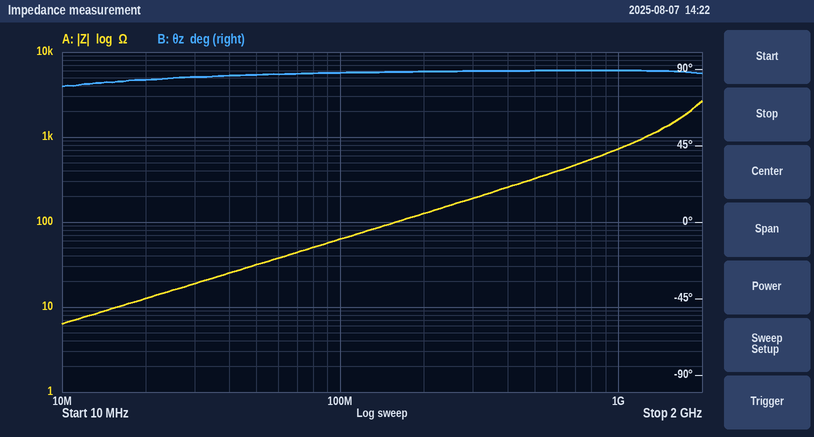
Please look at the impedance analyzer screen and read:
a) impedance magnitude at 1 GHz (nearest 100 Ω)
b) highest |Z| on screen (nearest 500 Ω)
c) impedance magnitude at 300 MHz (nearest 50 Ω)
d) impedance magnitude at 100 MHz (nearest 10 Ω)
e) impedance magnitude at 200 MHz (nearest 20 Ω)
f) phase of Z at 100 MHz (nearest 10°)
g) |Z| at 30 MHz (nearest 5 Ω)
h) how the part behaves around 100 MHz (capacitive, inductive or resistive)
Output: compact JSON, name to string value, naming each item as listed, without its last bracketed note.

{"impedance magnitude at 1 GHz": "700 Ω", "highest |Z| on screen": "2.5 kΩ", "impedance magnitude at 300 MHz": "200 Ω", "impedance magnitude at 100 MHz": "60 Ω", "impedance magnitude at 200 MHz": "120 Ω", "phase of Z at 100 MHz": "90°", "|Z| at 30 MHz": "20 Ω", "how the part behaves around 100 MHz": "inductive"}
